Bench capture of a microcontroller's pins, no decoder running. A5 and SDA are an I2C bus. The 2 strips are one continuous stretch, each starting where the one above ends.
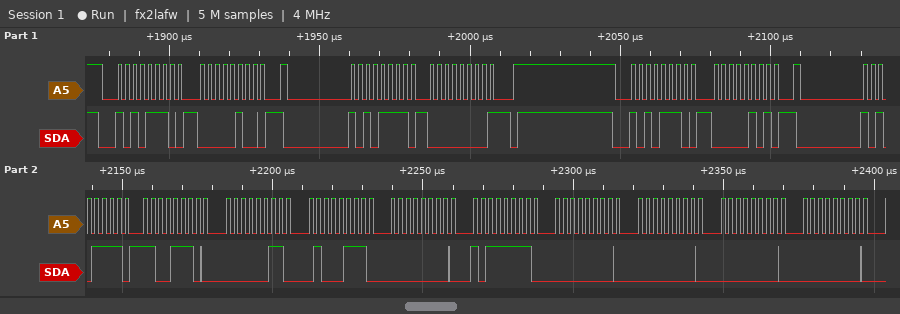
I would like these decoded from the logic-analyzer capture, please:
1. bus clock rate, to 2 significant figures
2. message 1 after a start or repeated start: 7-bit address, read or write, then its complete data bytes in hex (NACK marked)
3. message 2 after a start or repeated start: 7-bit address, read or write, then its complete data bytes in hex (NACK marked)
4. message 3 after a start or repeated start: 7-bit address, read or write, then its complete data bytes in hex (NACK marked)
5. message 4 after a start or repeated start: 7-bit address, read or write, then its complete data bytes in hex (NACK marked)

400 kHz
0x57 write: 04
0x57 read: 00 NACK
0x57 write: 05
0x57 read: CE 03 47 00 BF 00 00 00 00
